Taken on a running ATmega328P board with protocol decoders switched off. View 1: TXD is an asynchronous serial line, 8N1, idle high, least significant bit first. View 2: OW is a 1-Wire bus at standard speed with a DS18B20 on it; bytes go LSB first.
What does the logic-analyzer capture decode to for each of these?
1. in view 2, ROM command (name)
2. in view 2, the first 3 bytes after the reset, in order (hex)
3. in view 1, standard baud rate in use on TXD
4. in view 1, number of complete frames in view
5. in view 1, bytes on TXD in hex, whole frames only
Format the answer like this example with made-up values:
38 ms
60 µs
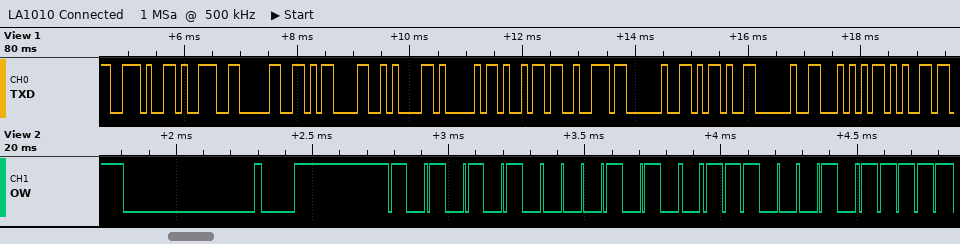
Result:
Match ROM
55 28 47
9600 baud
13
2E 39 30 0D 0A 41 69 72 20 2D 20 54 65
